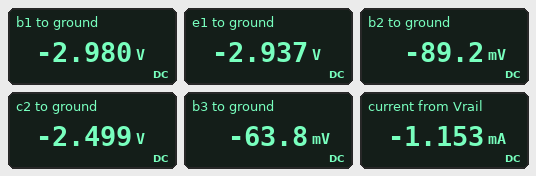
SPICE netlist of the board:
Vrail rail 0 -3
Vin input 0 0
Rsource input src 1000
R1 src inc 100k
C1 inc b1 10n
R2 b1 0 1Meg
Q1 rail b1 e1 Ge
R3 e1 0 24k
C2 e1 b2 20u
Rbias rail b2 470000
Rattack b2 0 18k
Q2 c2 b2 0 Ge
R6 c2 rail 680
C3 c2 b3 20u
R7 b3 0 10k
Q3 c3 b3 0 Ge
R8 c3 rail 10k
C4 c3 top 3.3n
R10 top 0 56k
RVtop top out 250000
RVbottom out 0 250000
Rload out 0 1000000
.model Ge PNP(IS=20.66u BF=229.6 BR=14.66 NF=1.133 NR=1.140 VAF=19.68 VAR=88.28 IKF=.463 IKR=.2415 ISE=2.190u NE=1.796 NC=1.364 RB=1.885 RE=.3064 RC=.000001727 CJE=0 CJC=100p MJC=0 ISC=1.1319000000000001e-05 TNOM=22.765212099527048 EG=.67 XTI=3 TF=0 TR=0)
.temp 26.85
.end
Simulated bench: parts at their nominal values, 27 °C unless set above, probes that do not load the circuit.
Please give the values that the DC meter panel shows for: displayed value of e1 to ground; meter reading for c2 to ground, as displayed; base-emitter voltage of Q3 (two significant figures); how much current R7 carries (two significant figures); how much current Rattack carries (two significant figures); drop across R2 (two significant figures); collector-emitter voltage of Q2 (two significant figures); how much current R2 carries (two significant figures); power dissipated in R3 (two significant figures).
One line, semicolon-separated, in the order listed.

-2.937 V; -2.499 V; -64 mV; 6.4 µA; 5.0 µA; 3.0 V; -2.5 V; 3.0 µA; 360 µW
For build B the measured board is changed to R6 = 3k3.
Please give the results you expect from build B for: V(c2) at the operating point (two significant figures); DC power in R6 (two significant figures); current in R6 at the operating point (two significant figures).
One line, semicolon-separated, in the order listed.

-760 mV; 1.5 mW; 680 µA
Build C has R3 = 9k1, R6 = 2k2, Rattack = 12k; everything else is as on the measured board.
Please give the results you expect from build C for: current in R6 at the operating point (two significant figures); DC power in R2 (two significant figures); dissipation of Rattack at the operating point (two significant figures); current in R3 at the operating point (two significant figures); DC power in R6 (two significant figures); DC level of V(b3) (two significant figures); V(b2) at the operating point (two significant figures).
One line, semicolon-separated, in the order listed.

610 µA; 8.7 µW; 600 nW; 320 µA; 820 µW; -64 mV; -85 mV
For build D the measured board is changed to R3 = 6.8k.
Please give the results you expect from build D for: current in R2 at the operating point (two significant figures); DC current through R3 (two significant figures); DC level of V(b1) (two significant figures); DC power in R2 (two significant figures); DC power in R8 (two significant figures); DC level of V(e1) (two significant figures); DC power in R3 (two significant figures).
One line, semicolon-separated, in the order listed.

2.9 µA; 420 µA; -2.9 V; 8.5 µW; 820 µW; -2.8 V; 1.2 mW
